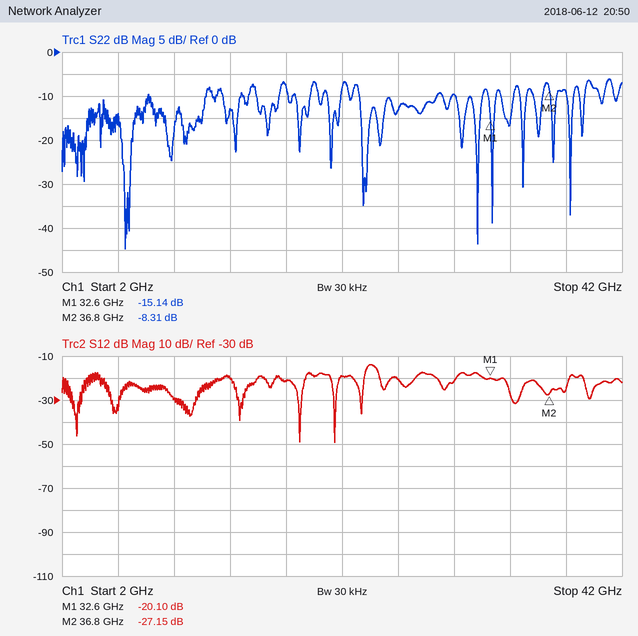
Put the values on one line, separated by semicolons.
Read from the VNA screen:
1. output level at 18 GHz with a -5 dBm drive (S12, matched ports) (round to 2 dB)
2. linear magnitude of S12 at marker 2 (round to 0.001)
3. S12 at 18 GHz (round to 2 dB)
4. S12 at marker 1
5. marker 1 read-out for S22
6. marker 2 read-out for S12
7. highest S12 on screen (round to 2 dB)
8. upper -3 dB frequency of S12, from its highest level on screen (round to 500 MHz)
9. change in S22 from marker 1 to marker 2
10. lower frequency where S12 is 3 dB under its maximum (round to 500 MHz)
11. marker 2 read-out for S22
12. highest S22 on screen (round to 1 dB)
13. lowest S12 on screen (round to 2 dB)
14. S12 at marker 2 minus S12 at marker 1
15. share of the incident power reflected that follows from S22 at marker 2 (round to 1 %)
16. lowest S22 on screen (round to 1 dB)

-26 dBm; 0.044; -22 dB; -20.10 dB; -15.14 dB; -27.15 dB; -14 dB; 24.5 GHz; 6.83 dB; 23.5 GHz; -8.31 dB; -6 dB; -50 dB; -7.05 dB; 15 %; -45 dB
